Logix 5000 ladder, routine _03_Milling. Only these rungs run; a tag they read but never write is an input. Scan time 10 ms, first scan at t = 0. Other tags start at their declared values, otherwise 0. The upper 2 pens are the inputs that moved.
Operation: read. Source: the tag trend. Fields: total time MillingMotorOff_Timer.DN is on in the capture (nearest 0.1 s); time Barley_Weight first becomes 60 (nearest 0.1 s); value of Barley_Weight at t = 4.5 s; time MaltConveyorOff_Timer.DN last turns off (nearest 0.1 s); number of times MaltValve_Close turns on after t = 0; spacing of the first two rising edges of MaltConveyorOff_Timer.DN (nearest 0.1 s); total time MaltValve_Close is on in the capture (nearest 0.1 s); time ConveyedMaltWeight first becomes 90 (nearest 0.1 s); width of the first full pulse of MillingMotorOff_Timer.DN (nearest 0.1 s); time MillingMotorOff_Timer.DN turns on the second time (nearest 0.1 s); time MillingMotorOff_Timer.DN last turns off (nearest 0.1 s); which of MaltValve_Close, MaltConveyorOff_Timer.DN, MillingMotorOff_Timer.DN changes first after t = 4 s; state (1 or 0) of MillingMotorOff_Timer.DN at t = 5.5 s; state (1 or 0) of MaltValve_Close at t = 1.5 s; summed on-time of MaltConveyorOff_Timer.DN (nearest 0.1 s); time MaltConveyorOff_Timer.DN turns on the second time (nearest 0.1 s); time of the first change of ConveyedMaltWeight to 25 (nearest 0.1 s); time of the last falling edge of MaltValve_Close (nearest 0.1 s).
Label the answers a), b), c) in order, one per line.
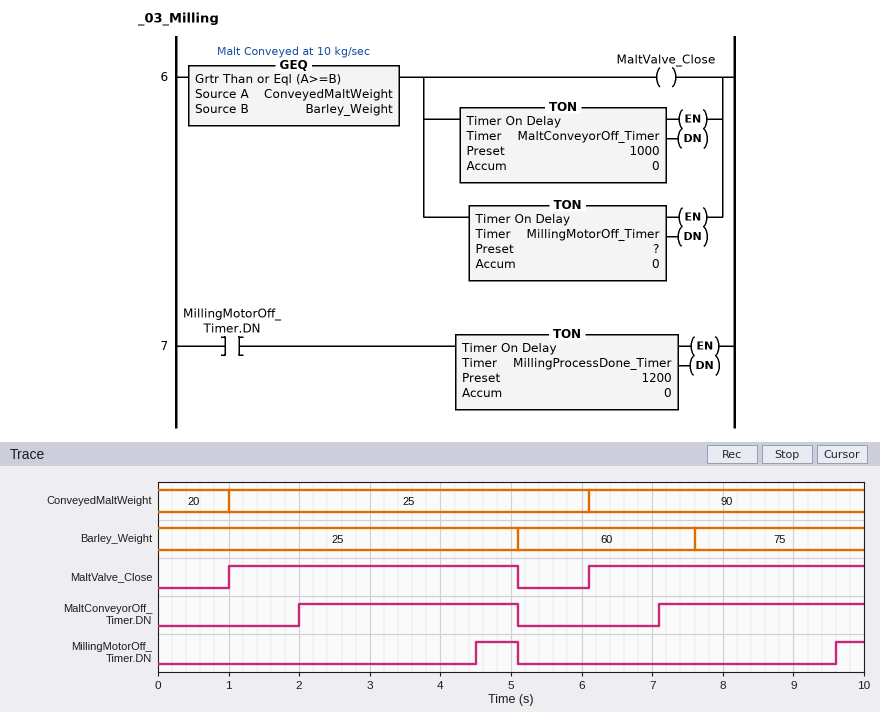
a) 1.0 s
b) 5.1 s
c) 25
d) 5.1 s
e) 2
f) 5.1 s
g) 8.0 s
h) 6.1 s
i) 0.6 s
j) 9.6 s
k) 5.1 s
l) MillingMotorOff_Timer.DN
m) 0
n) 1
o) 6.0 s
p) 7.1 s
q) 1.0 s
r) 5.1 s
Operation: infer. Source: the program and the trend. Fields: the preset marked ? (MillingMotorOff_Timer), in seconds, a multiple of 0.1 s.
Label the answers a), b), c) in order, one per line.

a) 3.5 s
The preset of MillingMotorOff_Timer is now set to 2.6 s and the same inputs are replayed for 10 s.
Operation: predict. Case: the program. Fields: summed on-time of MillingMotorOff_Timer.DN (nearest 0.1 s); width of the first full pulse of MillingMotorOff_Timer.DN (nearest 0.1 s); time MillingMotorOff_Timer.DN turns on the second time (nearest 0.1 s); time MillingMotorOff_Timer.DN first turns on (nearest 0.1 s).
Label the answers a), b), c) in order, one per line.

a) 2.8 s
b) 1.5 s
c) 8.7 s
d) 3.6 s
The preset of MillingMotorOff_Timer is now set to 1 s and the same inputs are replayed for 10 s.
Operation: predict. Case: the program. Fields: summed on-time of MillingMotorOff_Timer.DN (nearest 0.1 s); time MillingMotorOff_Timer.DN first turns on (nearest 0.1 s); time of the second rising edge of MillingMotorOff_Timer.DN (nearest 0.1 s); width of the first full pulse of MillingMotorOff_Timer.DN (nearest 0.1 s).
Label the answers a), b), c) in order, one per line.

a) 6.0 s
b) 2.0 s
c) 7.1 s
d) 3.1 s
